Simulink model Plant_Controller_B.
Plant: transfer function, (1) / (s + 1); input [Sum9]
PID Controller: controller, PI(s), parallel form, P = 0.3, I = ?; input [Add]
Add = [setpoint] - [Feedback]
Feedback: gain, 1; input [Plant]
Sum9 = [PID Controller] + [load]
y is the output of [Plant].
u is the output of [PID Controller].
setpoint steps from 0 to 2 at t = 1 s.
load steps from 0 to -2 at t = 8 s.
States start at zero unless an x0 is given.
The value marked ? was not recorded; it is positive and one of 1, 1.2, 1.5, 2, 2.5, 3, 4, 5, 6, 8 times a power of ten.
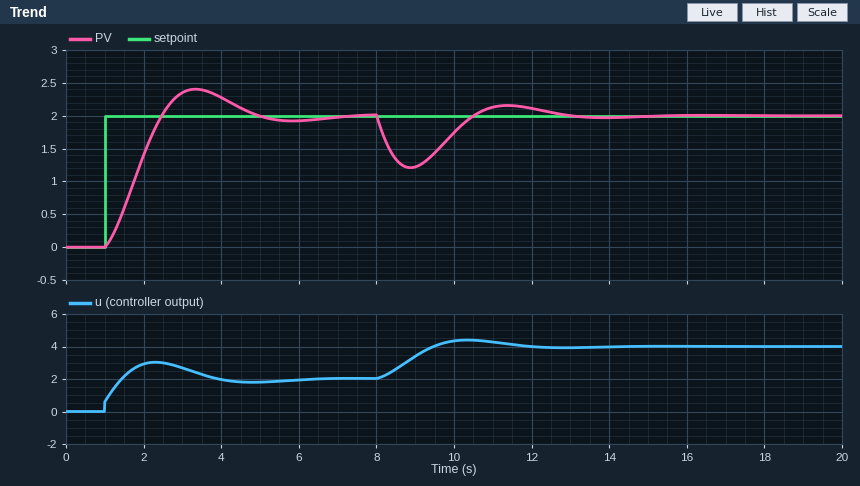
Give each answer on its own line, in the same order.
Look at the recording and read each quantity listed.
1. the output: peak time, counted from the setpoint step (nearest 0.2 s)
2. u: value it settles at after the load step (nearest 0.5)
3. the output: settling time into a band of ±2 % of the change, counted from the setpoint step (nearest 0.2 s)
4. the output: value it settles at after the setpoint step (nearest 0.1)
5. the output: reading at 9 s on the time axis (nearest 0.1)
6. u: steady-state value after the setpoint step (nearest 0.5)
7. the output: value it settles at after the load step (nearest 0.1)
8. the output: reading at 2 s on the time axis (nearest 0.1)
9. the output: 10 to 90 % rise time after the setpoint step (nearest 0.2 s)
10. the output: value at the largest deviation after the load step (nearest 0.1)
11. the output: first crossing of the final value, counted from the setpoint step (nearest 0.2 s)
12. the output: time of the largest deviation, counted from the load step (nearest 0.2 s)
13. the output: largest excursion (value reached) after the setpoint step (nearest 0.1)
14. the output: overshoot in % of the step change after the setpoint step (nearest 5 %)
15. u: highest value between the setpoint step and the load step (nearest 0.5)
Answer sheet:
2.4 s
4.0
5.8 s
2.0
1.2
2.0
2.0
1.4
1.0 s
1.2
1.4 s
0.8 s
2.4
20 %
3.0
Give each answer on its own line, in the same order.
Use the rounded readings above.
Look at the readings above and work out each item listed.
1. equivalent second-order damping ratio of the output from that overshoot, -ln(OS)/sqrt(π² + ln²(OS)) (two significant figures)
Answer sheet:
0.46
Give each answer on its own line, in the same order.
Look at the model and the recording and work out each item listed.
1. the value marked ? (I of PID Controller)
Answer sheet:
2
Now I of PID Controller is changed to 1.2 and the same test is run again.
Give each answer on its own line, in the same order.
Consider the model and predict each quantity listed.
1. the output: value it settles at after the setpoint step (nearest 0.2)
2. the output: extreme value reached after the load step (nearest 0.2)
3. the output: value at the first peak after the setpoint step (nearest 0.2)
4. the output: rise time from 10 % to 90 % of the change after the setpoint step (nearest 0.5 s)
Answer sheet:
2.0
1.0
2.2
1.5 s
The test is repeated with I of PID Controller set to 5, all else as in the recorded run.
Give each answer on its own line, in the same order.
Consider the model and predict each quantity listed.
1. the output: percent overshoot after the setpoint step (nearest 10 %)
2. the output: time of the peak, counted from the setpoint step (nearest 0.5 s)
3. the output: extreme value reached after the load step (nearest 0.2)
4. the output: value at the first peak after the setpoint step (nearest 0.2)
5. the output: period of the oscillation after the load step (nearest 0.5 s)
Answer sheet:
40 %
1.5 s
1.4
2.8
3.0 s
